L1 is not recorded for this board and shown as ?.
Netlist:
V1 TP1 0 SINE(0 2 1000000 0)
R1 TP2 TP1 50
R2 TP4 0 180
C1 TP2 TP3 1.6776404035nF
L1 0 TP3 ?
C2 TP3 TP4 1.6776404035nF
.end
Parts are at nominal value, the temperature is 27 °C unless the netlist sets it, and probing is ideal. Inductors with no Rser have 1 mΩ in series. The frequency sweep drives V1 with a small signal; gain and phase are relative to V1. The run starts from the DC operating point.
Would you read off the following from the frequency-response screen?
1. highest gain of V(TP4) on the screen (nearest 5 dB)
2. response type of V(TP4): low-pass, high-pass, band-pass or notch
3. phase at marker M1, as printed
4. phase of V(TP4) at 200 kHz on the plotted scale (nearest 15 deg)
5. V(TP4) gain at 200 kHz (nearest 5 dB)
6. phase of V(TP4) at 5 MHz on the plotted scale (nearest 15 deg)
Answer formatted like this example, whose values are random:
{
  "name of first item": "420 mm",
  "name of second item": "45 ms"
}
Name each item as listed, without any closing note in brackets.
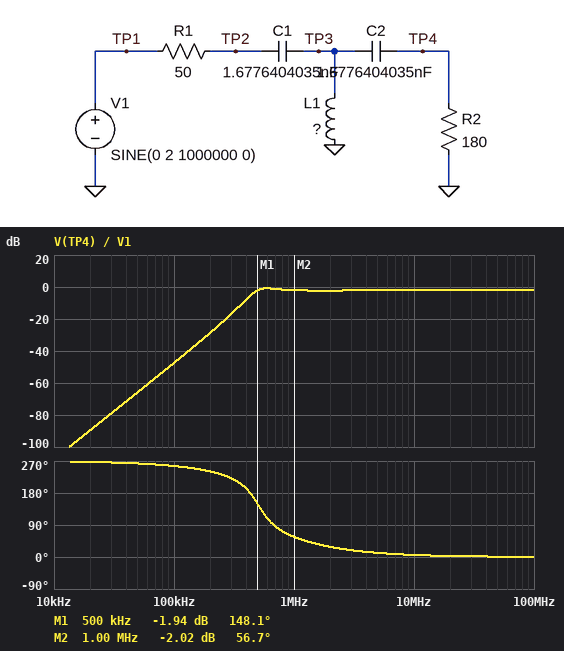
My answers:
{
  "highest gain of V(TP4) on the screen": "0 dB",
  "response type of V(TP4): low-pass, high-pass, band-pass or notch": "high-pass",
  "phase at marker M1, as printed": "148.1 deg",
  "phase of V(TP4) at 200 kHz on the plotted scale": "240 deg",
  "V(TP4) gain at 200 kHz": "-30 dB",
  "phase of V(TP4) at 5 MHz on the plotted scale": "15 deg"
}
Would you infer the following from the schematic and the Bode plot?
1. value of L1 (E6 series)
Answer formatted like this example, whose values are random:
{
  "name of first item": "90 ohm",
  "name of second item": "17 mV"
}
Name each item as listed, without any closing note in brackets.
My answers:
{
  "value of L1": "33 µH"
}
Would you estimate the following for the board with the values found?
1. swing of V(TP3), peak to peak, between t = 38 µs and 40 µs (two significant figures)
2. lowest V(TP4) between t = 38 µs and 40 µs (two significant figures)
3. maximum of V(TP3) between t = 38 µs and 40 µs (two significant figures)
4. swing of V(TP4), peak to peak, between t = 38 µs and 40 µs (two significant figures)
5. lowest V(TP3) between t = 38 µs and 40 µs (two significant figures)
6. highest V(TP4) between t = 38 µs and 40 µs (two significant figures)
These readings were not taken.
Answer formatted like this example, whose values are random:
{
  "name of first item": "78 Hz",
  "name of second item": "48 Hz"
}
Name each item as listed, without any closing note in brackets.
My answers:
{
  "swing of V(TP3), peak to peak, between t = 38 µs and 40 µs": "3.6 V",
  "lowest V(TP4) between t = 38 µs and 40 µs": "-1.6 V",
  "maximum of V(TP3) between t = 38 µs and 40 µs": "1.8 V",
  "swing of V(TP4), peak to peak, between t = 38 µs and 40 µs": "3.2 V",
  "lowest V(TP3) between t = 38 µs and 40 µs": "-1.8 V",
  "highest V(TP4) between t = 38 µs and 40 µs": "1.6 V"
}
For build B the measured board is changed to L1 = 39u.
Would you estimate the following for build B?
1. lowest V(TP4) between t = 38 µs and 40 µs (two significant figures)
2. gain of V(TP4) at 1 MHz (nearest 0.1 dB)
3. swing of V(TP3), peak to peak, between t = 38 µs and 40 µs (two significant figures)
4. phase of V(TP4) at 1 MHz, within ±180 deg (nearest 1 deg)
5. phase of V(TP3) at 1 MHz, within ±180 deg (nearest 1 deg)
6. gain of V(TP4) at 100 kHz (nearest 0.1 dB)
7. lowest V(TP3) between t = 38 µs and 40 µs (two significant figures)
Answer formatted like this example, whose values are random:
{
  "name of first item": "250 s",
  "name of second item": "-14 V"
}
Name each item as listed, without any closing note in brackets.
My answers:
{
  "lowest V(TP4) between t = 38 µs and 40 µs": "-1.5 V",
  "gain of V(TP4) at 1 MHz": "-2.4 dB",
  "swing of V(TP3), peak to peak, between t = 38 µs and 40 µs": "3.4 V",
  "phase of V(TP4) at 1 MHz, within ±180 deg": "53 deg",
  "phase of V(TP3) at 1 MHz, within ±180 deg": "26 deg",
  "gain of V(TP4) at 100 kHz": "-45.9 dB",
  "lowest V(TP3) between t = 38 µs and 40 µs": "-1.7 V"
}
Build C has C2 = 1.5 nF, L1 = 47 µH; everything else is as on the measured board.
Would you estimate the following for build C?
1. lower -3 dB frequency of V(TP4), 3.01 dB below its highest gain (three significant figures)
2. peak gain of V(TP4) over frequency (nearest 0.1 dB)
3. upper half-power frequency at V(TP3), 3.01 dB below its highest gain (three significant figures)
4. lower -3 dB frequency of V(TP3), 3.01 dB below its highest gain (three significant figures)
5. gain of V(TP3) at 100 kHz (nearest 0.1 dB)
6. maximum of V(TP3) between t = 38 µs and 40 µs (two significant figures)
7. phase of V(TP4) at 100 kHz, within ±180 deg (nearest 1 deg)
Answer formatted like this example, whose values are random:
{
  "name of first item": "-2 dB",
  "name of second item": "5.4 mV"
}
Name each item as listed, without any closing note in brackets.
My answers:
{
  "lower -3 dB frequency of V(TP4), 3.01 dB below its highest gain": "385 kHz",
  "peak gain of V(TP4) over frequency": "-0.9 dB",
  "upper half-power frequency at V(TP3), 3.01 dB below its highest gain": "636 kHz",
  "lower -3 dB frequency of V(TP3), 3.01 dB below its highest gain": "371 kHz",
  "gain of V(TP3) at 100 kHz": "-29.6 dB",
  "maximum of V(TP3) between t = 38 µs and 40 µs": "1.7 V",
  "phase of V(TP4) at 100 kHz, within ±180 deg": "-103 deg"
}
